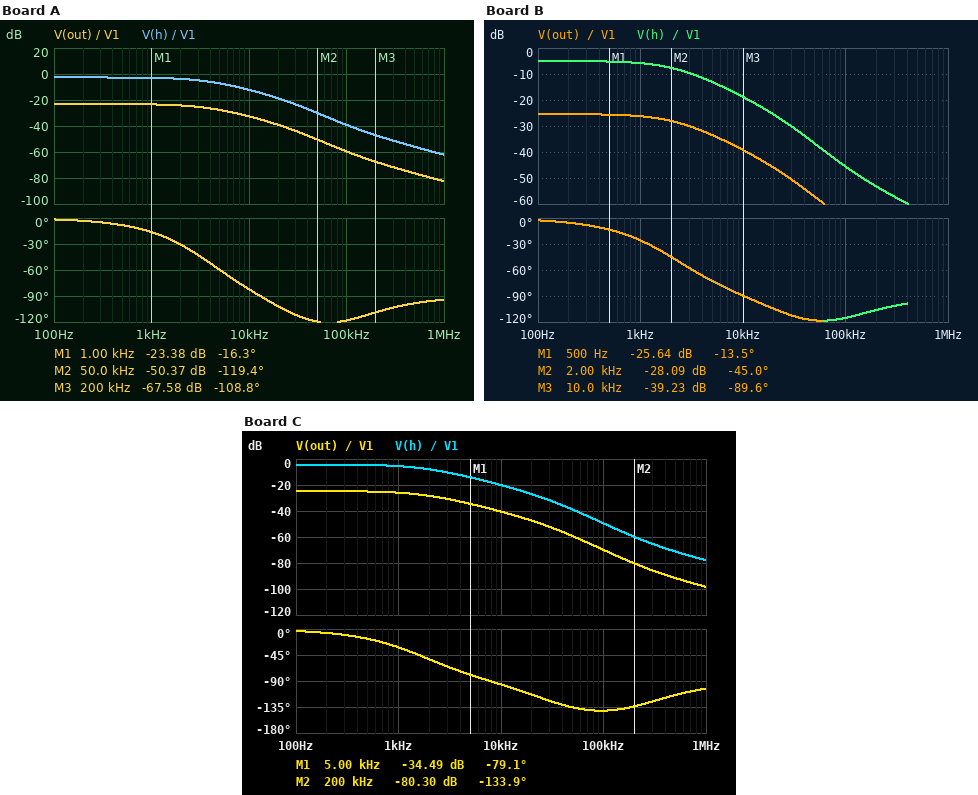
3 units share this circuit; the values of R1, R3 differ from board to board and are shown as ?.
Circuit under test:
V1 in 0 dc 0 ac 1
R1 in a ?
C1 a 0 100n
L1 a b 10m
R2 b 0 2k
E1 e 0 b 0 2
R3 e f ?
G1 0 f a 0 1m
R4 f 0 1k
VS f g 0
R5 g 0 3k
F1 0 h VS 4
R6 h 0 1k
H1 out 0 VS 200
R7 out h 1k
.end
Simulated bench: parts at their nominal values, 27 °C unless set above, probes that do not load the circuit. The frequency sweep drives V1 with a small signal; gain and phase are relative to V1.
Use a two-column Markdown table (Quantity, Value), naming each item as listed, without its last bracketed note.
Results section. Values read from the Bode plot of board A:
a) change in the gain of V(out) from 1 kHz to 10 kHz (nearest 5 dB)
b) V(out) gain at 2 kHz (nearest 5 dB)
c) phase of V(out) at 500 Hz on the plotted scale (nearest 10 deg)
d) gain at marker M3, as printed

| Quantity | Value |
|---|---|
| change in the gain of V(out) from 1 kHz to 10 kHz | -10 dB |
| V(out) gain at 2 kHz | -25 dB |
| phase of V(out) at 500 Hz on the plotted scale | -10 deg |
| gain at marker M3, as printed | -67.58 dB |
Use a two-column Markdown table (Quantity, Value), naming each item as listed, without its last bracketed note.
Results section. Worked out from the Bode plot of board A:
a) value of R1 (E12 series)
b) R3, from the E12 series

| Quantity | Value |
|---|---|
| value of R1 | 560 Ω |
| R3, from the E12 series | 820 Ω |
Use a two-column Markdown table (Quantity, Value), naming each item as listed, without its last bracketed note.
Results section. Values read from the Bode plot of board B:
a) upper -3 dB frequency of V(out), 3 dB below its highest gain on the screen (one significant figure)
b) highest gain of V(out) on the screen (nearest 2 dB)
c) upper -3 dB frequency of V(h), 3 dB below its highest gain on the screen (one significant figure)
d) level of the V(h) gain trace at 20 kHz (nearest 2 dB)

| Quantity | Value |
|---|---|
| upper -3 dB frequency of V(out), 3 dB below its highest gain on the screen | 2 kHz |
| highest gain of V(out) on the screen | -26 dB |
| upper -3 dB frequency of V(h), 3 dB below its highest gain on the screen | 2 kHz |
| level of the V(h) gain trace at 20 kHz | -26 dB |
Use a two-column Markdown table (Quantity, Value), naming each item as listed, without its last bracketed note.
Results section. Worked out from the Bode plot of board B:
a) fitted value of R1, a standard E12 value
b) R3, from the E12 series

| Quantity | Value |
|---|---|
| fitted value of R1, a standard E12 value | 1.2 kΩ |
| R3, from the E12 series | 1 kΩ |
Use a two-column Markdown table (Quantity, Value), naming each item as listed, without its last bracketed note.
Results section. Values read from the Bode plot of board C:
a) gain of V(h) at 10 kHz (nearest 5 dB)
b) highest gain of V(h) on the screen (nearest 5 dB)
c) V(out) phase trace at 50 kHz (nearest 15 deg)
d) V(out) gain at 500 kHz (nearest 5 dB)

| Quantity | Value |
|---|---|
| gain of V(h) at 10 kHz | -20 dB |
| highest gain of V(h) on the screen | -5 dB |
| V(out) phase trace at 50 kHz | -135 deg |
| V(out) gain at 500 kHz | -90 dB |
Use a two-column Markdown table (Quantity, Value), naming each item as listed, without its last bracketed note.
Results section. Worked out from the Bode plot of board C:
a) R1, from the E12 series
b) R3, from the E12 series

| Quantity | Value |
|---|---|
| R1, from the E12 series | 1.8 kΩ |
| R3, from the E12 series | 270 Ω |
